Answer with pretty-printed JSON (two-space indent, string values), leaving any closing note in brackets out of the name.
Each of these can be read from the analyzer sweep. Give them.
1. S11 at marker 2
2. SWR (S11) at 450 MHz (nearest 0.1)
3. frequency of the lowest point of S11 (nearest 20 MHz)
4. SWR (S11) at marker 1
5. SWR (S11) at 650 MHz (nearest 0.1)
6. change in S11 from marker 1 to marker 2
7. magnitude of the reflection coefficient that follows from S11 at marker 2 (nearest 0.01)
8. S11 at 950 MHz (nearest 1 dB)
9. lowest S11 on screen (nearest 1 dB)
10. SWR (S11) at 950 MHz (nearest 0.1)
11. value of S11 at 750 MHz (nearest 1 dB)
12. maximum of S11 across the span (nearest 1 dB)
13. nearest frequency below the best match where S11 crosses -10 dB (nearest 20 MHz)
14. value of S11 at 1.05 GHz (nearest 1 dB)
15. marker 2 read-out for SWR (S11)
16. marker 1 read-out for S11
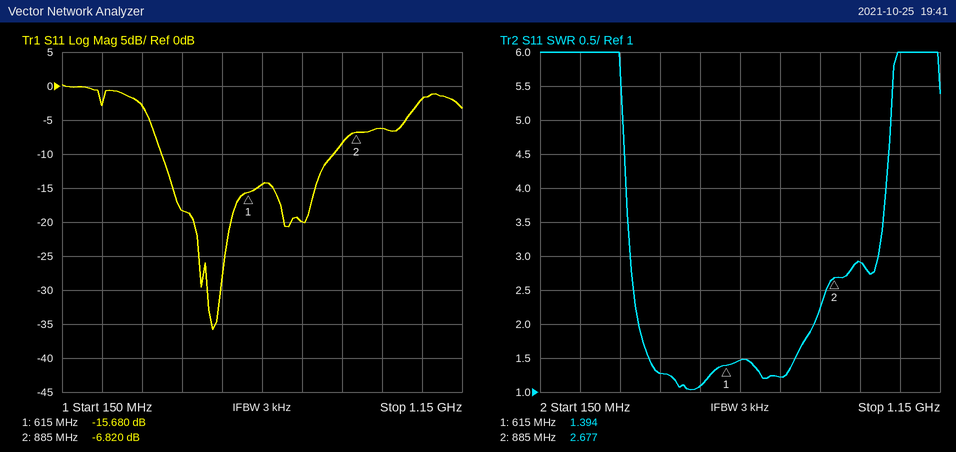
{
  "S11 at marker 2": "-6.820 dB",
  "SWR (S11) at 450 MHz": "1.3",
  "frequency of the lowest point of S11": "520 MHz",
  "SWR (S11) at marker 1": "1.394",
  "SWR (S11) at 650 MHz": "1.5",
  "change in S11 from marker 1 to marker 2": "8.860 dB",
  "magnitude of the reflection coefficient that follows from S11 at marker 2": "0.46",
  "S11 at 950 MHz": "-6 dB",
  "lowest S11 on screen": "-36 dB",
  "SWR (S11) at 950 MHz": "2.9",
  "value of S11 at 750 MHz": "-20 dB",
  "maximum of S11 across the span": "0 dB",
  "nearest frequency below the best match where S11 crosses -10 dB": "400 MHz",
  "value of S11 at 1.05 GHz": "-2 dB",
  "marker 2 read-out for SWR": "2.677",
  "marker 1 read-out for S11": "-15.680 dB"
}
